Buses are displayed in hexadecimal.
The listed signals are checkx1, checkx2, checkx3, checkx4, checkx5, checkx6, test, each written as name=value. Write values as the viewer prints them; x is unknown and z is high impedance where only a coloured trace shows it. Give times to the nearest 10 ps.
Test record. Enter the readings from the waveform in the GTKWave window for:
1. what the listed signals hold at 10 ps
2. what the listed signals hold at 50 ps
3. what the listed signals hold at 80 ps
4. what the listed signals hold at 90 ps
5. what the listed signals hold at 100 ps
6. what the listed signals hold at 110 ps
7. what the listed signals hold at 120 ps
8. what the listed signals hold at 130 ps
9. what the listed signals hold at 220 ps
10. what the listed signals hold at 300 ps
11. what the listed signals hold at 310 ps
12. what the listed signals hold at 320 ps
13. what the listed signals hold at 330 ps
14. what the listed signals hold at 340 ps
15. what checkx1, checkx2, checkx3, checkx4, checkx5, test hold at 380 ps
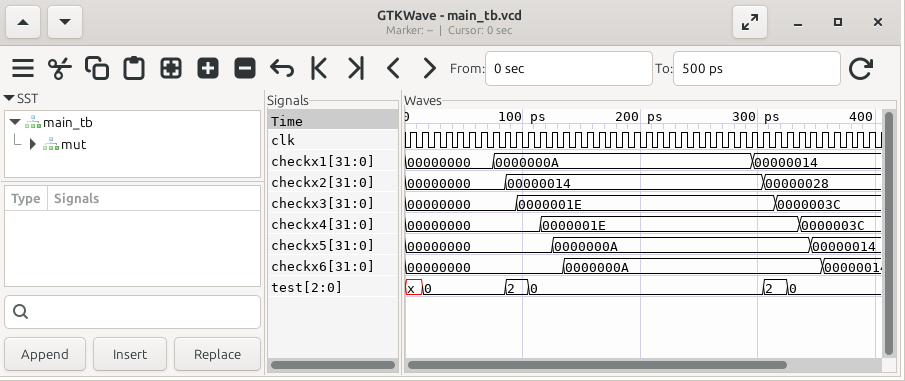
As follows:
checkx1=00000000, checkx2=00000000, checkx3=00000000, checkx4=00000000, checkx5=00000000, checkx6=00000000, test=x
checkx1=00000000, checkx2=00000000, checkx3=00000000, checkx4=00000000, checkx5=00000000, checkx6=00000000, test=0
checkx1=0000000A, checkx2=00000000, checkx3=00000000, checkx4=00000000, checkx5=00000000, checkx6=00000000, test=0
checkx1=0000000A, checkx2=00000014, checkx3=00000000, checkx4=00000000, checkx5=00000000, checkx6=00000000, test=2
checkx1=0000000A, checkx2=00000014, checkx3=0000001E, checkx4=00000000, checkx5=00000000, checkx6=00000000, test=2
checkx1=0000000A, checkx2=00000014, checkx3=0000001E, checkx4=00000000, checkx5=00000000, checkx6=00000000, test=0
checkx1=0000000A, checkx2=00000014, checkx3=0000001E, checkx4=0000001E, checkx5=00000000, checkx6=00000000, test=0
checkx1=0000000A, checkx2=00000014, checkx3=0000001E, checkx4=0000001E, checkx5=0000000A, checkx6=00000000, test=0
checkx1=0000000A, checkx2=00000014, checkx3=0000001E, checkx4=0000001E, checkx5=0000000A, checkx6=0000000A, test=0
checkx1=00000014, checkx2=00000014, checkx3=0000001E, checkx4=0000001E, checkx5=0000000A, checkx6=0000000A, test=0
checkx1=00000014, checkx2=00000028, checkx3=0000001E, checkx4=0000001E, checkx5=0000000A, checkx6=0000000A, test=2
checkx1=00000014, checkx2=00000028, checkx3=0000003C, checkx4=0000001E, checkx5=0000000A, checkx6=0000000A, test=2
checkx1=00000014, checkx2=00000028, checkx3=0000003C, checkx4=0000001E, checkx5=0000000A, checkx6=0000000A, test=0
checkx1=00000014, checkx2=00000028, checkx3=0000003C, checkx4=0000003C, checkx5=0000000A, checkx6=0000000A, test=0
checkx1=00000014, checkx2=00000028, checkx3=0000003C, checkx4=0000003C, checkx5=00000014, test=0
